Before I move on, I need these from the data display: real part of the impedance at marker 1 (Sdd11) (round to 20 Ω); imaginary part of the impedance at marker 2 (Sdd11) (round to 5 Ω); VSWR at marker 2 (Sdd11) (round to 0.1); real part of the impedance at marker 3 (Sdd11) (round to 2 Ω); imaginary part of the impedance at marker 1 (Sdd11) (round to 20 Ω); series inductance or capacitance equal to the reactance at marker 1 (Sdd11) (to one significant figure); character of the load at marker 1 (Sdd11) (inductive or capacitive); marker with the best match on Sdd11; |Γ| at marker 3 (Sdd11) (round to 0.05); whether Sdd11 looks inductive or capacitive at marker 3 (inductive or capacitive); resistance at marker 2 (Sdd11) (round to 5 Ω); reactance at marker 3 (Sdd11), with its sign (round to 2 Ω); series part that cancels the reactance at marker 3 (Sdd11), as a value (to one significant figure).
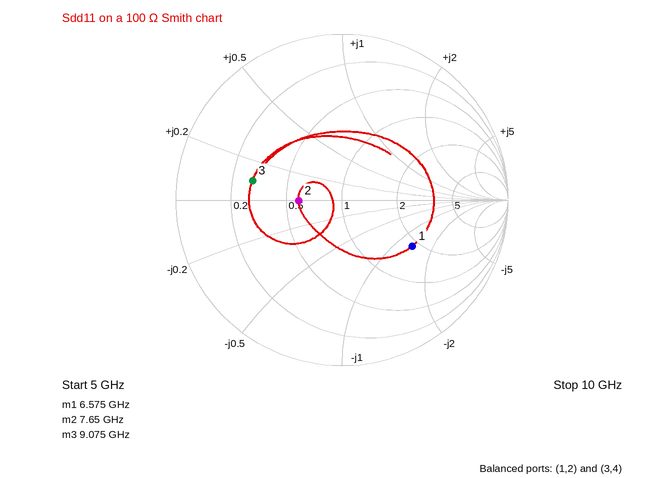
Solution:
180 Ω
0 Ω
1.7
30 Ω
-140 Ω
200 fF
capacitive
marker 2
0.55
inductive
60 Ω
+10 Ω
2 pF
